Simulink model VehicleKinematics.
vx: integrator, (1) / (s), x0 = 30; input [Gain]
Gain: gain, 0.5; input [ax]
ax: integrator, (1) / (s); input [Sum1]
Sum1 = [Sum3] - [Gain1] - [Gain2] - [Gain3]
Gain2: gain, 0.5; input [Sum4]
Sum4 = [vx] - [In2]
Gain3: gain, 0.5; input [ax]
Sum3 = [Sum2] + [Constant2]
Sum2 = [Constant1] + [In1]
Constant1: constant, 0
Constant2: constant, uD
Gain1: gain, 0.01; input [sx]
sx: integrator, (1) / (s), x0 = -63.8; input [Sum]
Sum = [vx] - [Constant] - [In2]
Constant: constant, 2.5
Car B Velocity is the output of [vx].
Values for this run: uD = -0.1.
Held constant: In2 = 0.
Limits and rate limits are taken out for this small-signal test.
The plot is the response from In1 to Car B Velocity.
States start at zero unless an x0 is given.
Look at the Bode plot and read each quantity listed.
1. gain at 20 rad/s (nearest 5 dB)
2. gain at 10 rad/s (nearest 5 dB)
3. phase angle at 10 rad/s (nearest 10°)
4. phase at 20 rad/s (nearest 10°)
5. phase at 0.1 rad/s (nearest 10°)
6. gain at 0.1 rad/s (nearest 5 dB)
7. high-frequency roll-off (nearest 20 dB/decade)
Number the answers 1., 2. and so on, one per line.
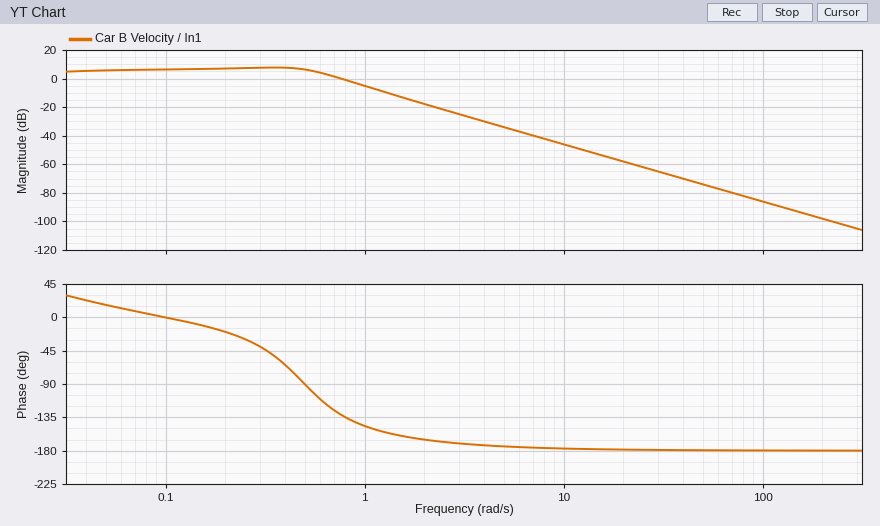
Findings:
1. -60 dB
2. -45 dB
3. -180°
4. -180°
5. 0°
6. 5 dB
7. -40 dB/decade
